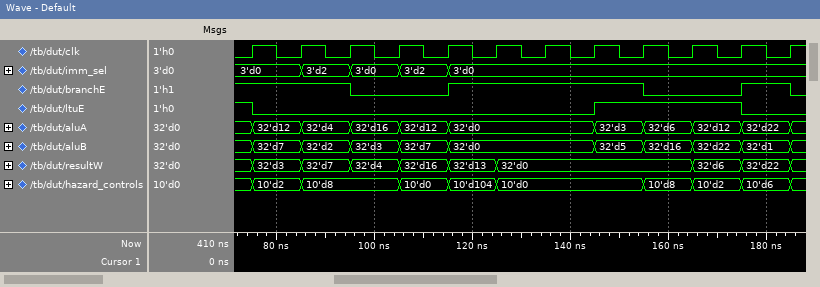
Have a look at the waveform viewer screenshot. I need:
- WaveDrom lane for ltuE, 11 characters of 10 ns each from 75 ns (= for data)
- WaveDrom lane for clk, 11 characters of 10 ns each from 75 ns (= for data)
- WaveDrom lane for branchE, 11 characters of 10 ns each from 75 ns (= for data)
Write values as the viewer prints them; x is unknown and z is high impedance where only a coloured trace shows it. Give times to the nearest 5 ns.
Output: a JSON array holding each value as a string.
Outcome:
["{name: 'ltuE', wave: '0......1..0'}", "{name: 'clk', wave: 'p..........'}", "{name: 'branchE', wave: '1.0.1...0.1'}"]
